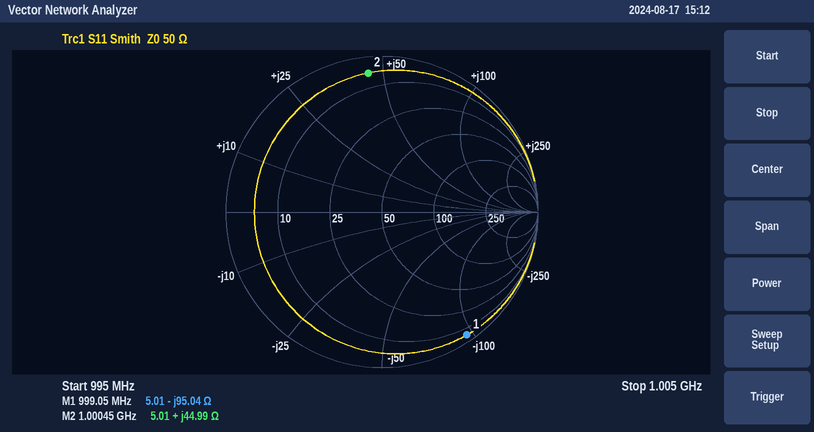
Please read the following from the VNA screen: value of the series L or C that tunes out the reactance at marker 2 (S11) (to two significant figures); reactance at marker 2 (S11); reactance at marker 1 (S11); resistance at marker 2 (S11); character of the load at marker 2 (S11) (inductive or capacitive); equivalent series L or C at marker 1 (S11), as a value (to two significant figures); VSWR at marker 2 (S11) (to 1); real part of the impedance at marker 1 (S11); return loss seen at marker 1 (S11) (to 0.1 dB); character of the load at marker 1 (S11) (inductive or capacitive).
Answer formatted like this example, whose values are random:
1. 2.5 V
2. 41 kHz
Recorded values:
1. 3.5 pF
2. +44.99 Ω
3. -95.04 Ω
4. 5.01 Ω
5. inductive
6. 1.7 pF
7. 18
8. 5.01 Ω
9. 0.4 dB
10. capacitive
